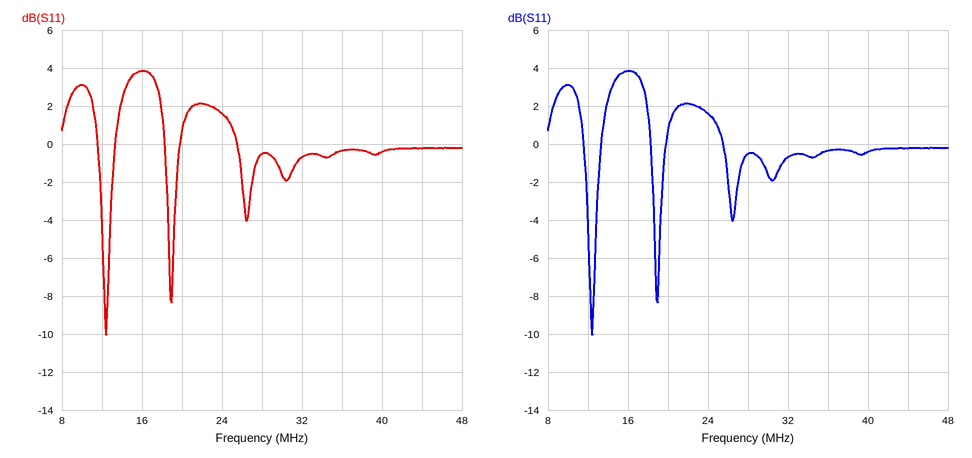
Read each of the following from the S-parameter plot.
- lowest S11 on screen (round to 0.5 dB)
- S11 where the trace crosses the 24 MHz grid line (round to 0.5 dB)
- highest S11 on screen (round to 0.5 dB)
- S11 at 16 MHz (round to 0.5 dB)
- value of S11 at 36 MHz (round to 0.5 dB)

-10.0 dB
1.5 dB
4.0 dB
4.0 dB
-0.5 dB
